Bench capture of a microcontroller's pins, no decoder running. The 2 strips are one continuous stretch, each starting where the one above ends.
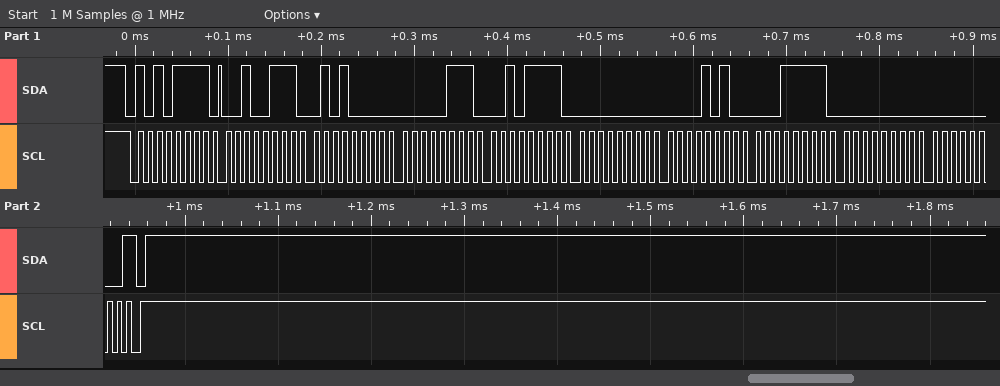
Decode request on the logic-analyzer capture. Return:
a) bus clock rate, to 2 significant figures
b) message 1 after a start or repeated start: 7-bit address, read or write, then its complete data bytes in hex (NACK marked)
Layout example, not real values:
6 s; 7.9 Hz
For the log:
100 kHz; 0x57 read: 27 50 07 2F 00 0A 1F 00 00 NACK
